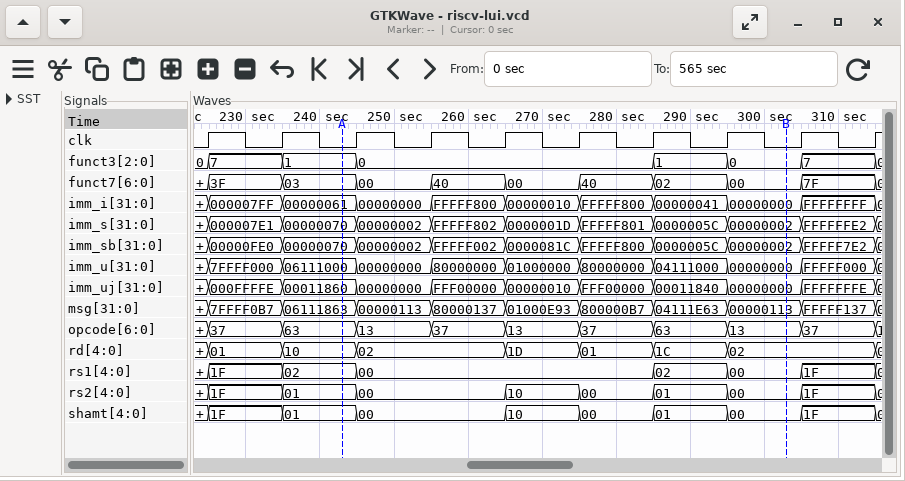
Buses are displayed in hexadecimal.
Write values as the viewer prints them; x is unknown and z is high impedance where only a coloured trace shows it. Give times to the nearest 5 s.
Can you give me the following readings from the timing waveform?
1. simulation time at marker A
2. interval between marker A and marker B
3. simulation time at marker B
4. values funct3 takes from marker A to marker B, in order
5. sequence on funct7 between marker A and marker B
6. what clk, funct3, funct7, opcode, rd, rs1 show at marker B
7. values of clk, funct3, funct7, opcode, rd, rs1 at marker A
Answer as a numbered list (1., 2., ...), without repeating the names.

1. 245 s
2. 60 s
3. 305 s
4. 1, 0, 1, 0
5. 03, 00, 40, 00, 40, 02, 00
6. clk=0, funct3=0, funct7=00, opcode=13, rd=02, rs1=00
7. clk=0, funct3=1, funct7=03, opcode=63, rd=10, rs1=02
